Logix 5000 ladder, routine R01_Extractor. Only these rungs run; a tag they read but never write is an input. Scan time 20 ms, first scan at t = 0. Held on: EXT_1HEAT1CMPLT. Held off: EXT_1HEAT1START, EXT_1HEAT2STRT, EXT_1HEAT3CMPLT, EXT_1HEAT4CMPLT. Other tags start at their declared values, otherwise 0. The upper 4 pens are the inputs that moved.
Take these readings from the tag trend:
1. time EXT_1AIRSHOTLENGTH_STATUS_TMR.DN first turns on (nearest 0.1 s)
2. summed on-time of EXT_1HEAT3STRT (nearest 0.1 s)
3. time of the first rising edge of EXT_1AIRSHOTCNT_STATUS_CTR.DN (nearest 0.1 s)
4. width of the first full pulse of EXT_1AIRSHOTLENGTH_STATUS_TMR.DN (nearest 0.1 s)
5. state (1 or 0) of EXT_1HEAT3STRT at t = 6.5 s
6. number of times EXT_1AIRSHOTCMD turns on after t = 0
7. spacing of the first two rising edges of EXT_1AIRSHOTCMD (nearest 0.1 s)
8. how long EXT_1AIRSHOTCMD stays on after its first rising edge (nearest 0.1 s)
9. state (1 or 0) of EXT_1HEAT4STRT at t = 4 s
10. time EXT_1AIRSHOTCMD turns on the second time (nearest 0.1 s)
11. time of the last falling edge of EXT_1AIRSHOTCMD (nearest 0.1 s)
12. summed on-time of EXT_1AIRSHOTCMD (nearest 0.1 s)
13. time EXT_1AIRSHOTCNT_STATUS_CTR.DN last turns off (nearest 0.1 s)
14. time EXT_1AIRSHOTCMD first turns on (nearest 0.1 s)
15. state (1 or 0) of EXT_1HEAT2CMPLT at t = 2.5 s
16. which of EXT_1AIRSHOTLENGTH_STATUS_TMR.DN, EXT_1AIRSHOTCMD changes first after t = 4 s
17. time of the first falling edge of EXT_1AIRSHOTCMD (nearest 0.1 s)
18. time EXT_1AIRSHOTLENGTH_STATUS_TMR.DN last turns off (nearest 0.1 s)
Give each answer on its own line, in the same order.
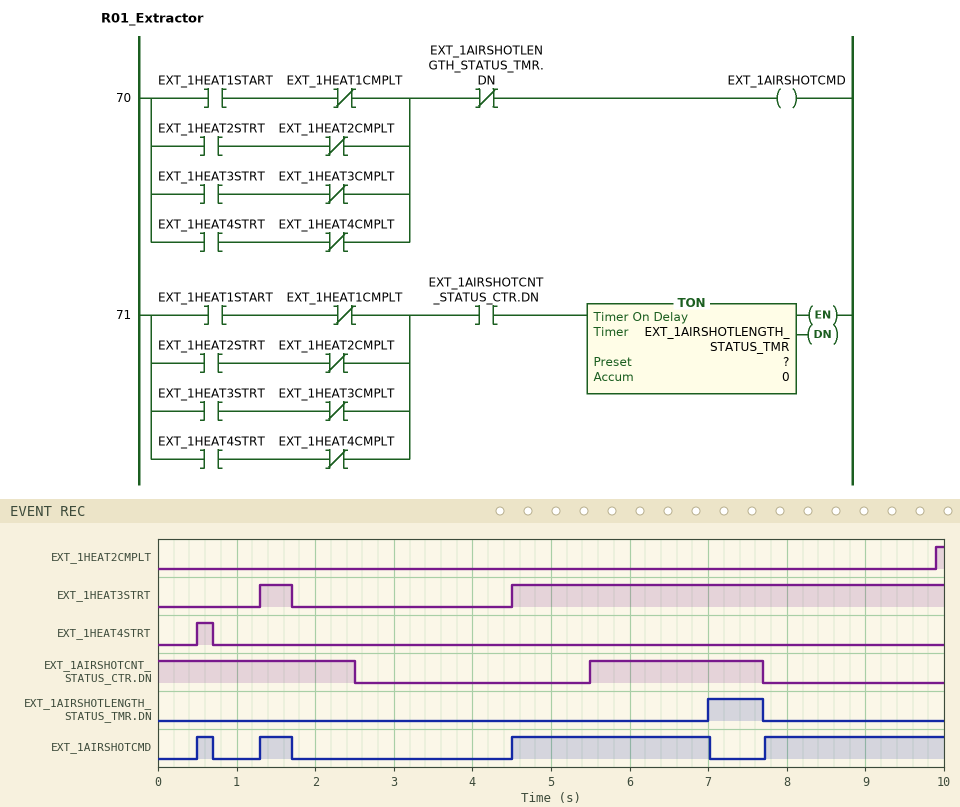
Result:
7.0 s
5.9 s
5.5 s
0.7 s
1
4
0.8 s
0.2 s
0
1.3 s
7.0 s
5.4 s
7.7 s
0.5 s
0
EXT_1AIRSHOTCMD
0.7 s
7.7 s
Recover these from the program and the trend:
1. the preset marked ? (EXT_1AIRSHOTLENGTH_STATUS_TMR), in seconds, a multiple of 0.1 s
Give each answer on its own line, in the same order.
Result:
1.5 s
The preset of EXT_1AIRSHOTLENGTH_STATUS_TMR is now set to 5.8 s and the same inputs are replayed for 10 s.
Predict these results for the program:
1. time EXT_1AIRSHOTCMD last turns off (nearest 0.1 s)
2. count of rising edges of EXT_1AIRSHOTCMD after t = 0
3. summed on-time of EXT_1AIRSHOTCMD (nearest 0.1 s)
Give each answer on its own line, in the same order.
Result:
1.7 s
3
6.1 s
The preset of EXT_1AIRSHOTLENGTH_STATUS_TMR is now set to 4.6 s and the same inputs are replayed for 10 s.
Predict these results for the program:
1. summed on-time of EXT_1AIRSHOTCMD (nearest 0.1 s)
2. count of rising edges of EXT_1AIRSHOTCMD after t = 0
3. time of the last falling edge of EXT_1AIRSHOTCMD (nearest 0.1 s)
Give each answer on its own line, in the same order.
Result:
6.1 s
3
1.7 s
